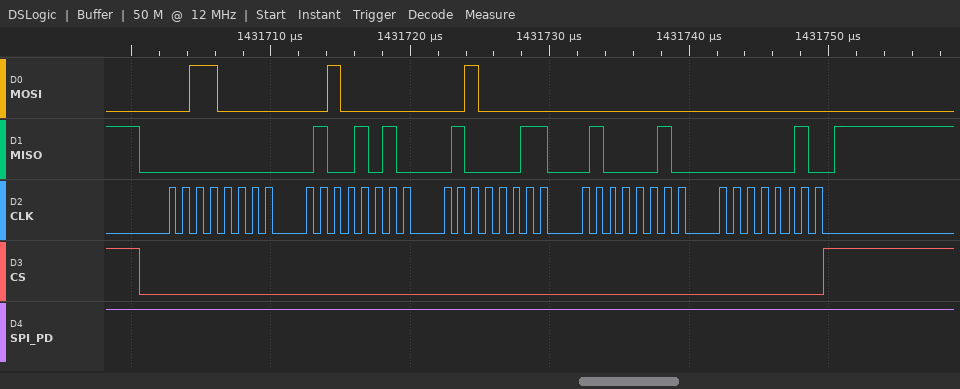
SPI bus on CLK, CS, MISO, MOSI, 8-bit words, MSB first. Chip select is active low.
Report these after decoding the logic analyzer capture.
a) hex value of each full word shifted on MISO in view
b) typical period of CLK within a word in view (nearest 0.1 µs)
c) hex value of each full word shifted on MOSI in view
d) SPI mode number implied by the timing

00, 4A, 43, 42, 02
1 µs
30, 20, 20, 00, 00
0
